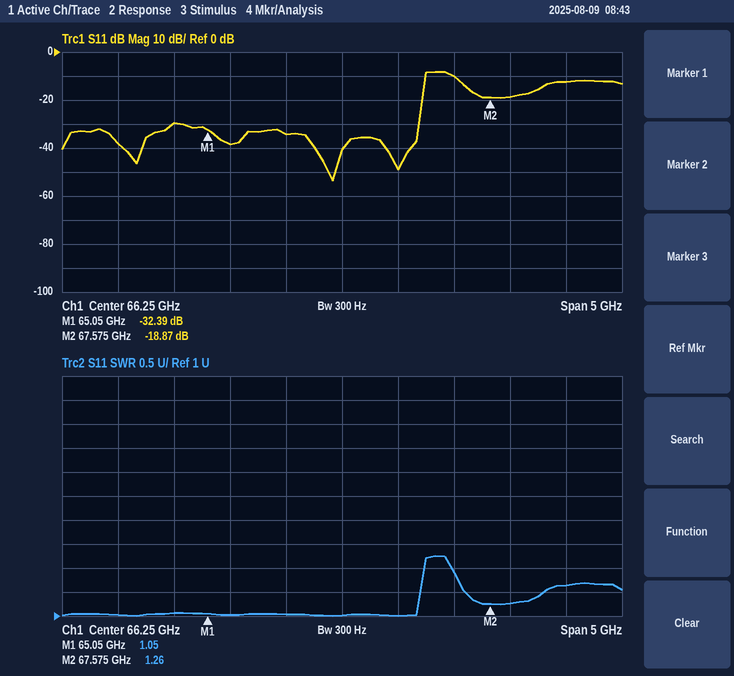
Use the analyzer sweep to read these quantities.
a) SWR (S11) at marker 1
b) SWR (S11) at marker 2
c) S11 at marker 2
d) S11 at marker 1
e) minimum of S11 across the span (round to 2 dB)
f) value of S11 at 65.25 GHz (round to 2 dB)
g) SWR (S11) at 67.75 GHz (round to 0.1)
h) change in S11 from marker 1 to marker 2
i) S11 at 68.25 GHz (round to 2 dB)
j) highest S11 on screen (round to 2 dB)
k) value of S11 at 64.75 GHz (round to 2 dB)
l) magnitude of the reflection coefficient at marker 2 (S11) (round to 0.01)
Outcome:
1.05
1.26
-18.87 dB
-32.39 dB
-54 dB
-38 dB
1.3
13.52 dB
-12 dB
-8 dB
-30 dB
0.11
